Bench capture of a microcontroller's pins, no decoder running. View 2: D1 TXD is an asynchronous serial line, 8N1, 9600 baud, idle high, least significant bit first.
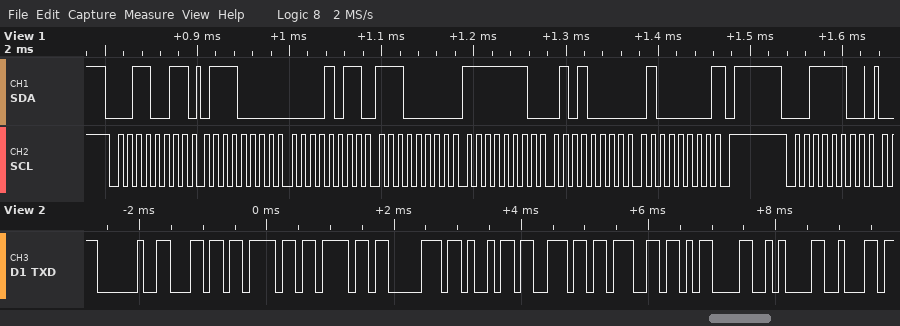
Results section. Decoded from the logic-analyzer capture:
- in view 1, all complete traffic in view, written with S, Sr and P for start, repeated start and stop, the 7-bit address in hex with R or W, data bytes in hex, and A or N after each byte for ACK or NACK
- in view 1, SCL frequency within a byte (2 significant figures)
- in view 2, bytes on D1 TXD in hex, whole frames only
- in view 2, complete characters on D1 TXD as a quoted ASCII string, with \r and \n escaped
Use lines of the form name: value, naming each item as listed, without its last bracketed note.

in view 1, all complete traffic in view, written with S, Sr and P for start, repeated start and stop, the 7-bit address in hex with R or W, data bytes in hex, and A or N after each byte for ACK or NACK: S 19R A 70 A 0B A E0 A FE A 50 A 40 N P S 1EW A
in view 1, SCL frequency within a byte: 100 kHz
in view 2, bytes on D1 TXD in hex, whole frames only: 20 6C 6F 6F 70 69 6E 67 0D 0A 62
in view 2, complete characters on D1 TXD as a quoted ASCII string, with \r and \n escaped: " looping\r\nb"
